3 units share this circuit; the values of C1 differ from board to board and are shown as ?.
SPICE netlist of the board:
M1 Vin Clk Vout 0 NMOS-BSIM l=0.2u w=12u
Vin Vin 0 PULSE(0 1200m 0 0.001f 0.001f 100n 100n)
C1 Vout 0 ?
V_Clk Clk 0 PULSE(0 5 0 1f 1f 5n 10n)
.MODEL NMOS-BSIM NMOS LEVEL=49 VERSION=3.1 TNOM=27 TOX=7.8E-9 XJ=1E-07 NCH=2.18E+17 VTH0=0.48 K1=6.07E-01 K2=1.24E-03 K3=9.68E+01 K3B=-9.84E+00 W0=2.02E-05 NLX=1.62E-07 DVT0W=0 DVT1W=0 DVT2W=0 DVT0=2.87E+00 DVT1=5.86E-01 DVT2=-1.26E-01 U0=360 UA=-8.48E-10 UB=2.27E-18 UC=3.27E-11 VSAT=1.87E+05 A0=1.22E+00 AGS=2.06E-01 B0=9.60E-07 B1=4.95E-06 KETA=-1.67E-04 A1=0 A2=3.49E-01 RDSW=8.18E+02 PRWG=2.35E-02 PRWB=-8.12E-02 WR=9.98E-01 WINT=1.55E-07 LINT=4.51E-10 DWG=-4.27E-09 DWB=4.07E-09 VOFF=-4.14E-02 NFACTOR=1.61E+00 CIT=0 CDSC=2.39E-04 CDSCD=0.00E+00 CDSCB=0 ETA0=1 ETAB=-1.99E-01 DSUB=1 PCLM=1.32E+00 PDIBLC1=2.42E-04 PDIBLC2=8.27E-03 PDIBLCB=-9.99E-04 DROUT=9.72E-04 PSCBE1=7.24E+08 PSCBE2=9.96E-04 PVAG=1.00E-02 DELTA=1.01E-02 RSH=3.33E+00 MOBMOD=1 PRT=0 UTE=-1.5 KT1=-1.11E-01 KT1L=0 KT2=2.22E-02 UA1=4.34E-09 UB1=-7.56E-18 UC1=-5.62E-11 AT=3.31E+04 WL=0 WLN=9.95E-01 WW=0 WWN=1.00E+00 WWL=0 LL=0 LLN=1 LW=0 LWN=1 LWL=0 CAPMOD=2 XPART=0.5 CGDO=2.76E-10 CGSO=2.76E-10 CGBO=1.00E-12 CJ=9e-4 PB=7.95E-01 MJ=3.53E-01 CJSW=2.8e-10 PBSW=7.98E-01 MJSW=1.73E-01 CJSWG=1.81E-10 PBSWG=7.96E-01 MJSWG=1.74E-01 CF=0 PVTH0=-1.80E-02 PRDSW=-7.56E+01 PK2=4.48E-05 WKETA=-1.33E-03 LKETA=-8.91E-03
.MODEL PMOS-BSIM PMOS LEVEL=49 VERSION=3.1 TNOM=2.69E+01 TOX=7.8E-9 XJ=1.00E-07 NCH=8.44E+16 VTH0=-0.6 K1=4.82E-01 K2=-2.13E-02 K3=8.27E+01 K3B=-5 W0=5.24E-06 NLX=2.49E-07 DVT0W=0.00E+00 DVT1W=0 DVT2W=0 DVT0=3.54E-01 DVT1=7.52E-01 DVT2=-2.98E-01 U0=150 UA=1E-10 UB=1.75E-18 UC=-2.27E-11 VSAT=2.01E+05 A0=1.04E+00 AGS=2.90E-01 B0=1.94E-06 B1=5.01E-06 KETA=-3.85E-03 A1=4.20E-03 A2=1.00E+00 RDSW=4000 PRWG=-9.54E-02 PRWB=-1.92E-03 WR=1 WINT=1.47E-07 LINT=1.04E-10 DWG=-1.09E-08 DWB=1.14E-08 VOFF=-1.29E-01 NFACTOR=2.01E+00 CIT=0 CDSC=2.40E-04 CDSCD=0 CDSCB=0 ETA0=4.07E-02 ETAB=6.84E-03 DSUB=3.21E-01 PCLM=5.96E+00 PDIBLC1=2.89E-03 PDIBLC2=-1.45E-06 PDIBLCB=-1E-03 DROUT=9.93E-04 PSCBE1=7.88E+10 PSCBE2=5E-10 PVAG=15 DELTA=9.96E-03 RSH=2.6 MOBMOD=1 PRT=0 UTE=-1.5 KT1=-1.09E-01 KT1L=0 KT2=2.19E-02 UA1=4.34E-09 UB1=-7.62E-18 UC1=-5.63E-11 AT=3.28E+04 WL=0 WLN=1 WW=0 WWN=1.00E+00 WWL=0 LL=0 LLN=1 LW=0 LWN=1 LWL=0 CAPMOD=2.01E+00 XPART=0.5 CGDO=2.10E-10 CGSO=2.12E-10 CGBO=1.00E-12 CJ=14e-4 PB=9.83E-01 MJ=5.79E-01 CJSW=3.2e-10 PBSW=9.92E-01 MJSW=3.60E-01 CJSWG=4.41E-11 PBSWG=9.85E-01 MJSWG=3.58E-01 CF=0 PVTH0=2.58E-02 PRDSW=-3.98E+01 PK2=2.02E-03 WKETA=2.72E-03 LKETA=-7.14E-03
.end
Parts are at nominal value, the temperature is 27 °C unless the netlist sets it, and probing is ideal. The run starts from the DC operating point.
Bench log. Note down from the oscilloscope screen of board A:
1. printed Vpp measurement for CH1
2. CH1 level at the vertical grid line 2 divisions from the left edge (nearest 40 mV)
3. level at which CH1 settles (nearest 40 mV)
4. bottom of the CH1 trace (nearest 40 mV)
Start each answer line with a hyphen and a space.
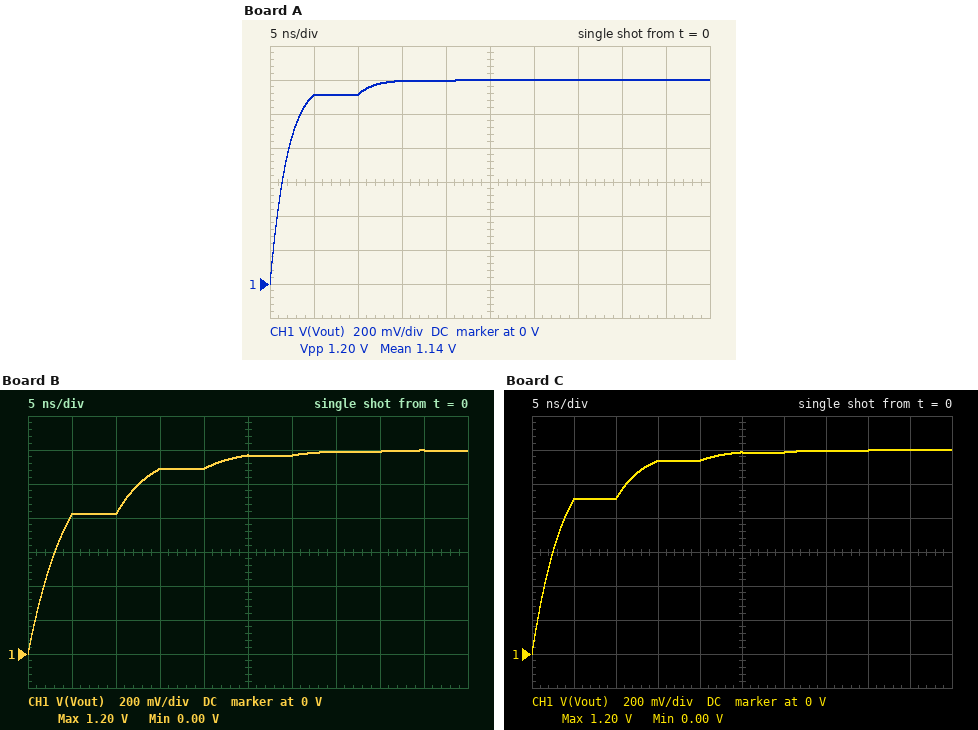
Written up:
- 1.20 V
- 1.12 V
- 1.20 V
- 0 V
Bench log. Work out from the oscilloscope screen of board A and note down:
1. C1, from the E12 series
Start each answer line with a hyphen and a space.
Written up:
- 15 pF
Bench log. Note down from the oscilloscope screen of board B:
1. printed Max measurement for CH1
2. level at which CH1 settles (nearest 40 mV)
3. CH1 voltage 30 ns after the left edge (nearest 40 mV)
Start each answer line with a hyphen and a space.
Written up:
- 1.20 V
- 1.20 V
- 1.16 V
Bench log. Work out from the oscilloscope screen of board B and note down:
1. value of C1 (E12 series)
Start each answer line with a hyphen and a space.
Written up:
- 33 pF
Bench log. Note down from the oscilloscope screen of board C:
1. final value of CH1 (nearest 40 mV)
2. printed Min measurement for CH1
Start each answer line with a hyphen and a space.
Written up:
- 1.20 V
- 0.00 V
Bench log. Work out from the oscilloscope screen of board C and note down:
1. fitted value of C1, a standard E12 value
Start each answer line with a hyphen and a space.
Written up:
- 27 pF
